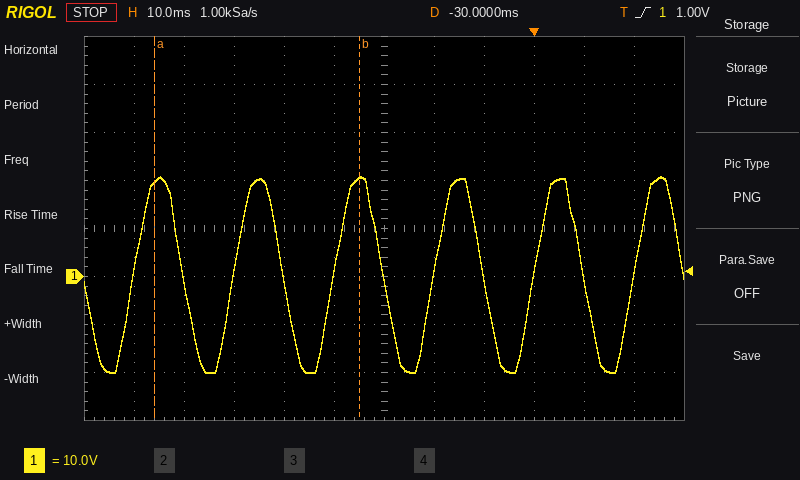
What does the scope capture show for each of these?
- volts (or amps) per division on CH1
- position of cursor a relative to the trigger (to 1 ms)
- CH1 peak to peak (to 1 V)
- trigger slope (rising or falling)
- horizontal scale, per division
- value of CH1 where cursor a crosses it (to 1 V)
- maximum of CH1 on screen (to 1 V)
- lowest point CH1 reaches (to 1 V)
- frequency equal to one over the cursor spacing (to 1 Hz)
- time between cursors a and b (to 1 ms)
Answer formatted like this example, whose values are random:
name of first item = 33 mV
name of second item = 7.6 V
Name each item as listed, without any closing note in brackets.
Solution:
volts (or amps) per division on CH1 = 10 V
position of cursor a relative to the trigger = -76 ms
CH1 peak to peak = 41 V
trigger slope = rising
horizontal scale, per division = 10 ms
value of CH1 where cursor a crosses it = 20 V
maximum of CH1 on screen = 21 V
lowest point CH1 reaches = -20 V
frequency equal to one over the cursor spacing = 24 Hz
time between cursors a and b = 41 ms
